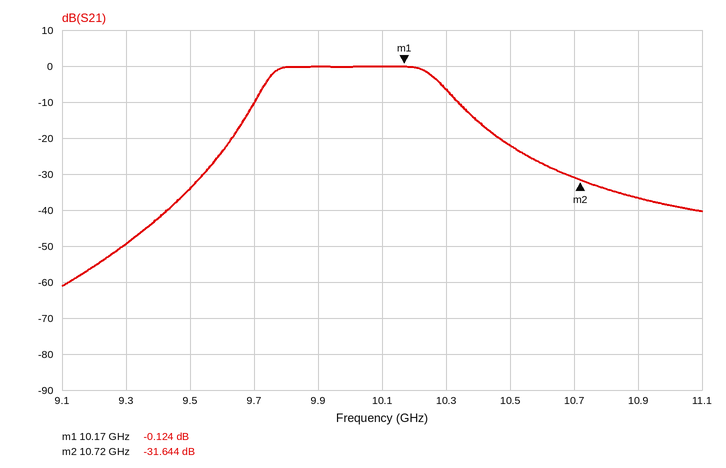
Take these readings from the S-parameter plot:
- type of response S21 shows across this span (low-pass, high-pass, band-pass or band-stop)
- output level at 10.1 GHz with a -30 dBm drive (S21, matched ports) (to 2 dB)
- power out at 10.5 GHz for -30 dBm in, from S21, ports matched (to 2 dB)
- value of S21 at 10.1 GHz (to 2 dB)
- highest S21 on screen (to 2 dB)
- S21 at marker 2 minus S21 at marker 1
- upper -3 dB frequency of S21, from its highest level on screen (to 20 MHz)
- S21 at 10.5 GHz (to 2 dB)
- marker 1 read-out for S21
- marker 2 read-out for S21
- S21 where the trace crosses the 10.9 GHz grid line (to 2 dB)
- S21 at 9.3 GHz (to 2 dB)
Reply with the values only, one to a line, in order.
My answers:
band-pass
-30 dBm
-52 dBm
0 dB
0 dB
-31.520 dB
10.26 GHz
-22 dB
-0.124 dB
-31.644 dB
-36 dB
-50 dB
